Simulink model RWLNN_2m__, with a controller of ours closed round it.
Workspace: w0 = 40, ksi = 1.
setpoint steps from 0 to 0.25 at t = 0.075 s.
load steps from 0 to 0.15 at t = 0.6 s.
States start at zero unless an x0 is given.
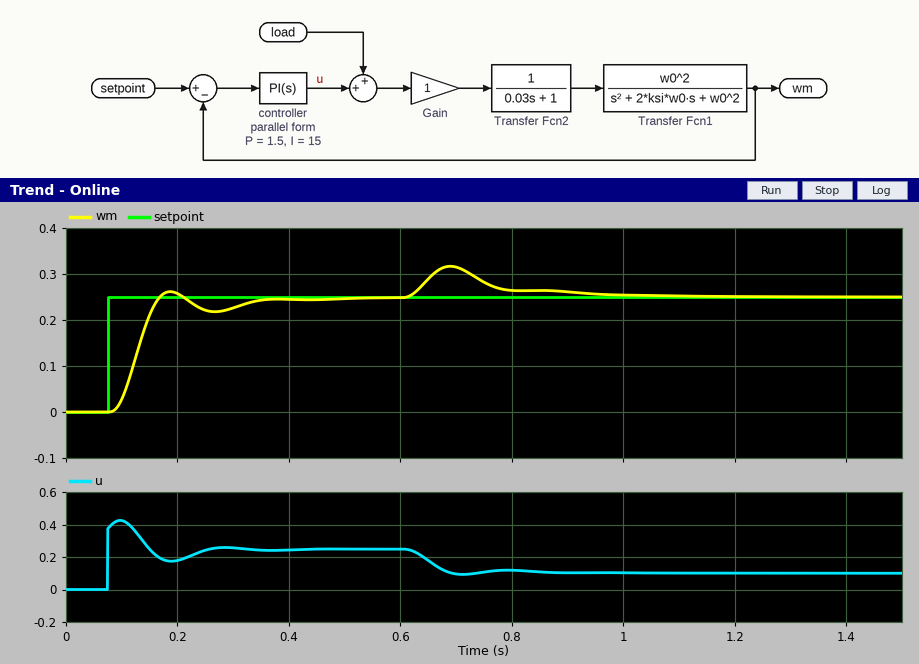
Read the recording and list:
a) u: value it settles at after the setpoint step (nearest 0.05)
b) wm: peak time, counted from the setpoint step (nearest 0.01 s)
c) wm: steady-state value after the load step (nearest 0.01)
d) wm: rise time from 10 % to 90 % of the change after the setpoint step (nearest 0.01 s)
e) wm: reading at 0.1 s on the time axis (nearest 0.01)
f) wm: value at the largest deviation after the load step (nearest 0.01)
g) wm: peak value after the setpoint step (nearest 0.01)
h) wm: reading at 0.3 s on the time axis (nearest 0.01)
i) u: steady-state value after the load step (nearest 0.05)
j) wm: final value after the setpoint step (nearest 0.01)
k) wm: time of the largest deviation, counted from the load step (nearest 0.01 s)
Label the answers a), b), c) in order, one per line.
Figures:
a) 0.25
b) 0.11 s
c) 0.25
d) 0.06 s
e) 0.03
f) 0.32
g) 0.26
h) 0.23
i) 0.10
j) 0.25
k) 0.09 s
